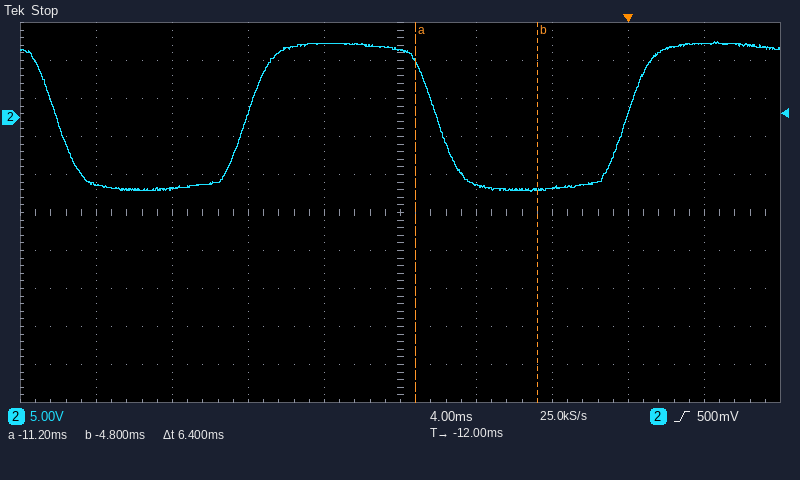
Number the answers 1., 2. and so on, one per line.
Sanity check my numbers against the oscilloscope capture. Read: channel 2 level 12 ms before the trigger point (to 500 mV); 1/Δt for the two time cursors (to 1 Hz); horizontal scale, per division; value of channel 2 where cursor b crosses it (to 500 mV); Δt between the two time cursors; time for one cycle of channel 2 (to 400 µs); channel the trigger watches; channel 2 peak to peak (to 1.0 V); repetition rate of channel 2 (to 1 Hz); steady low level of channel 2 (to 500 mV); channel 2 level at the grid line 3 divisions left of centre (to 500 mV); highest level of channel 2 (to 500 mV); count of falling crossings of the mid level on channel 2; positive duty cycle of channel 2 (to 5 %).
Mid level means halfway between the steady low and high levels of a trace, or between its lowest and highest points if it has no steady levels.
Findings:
1. 9.0 V
2. 156 Hz
3. 4 ms
4. -9.5 V
5. 6.4 ms
6. 20.0 ms
7. channel 2
8. 20.0 V
9. 50 Hz
10. -9.5 V
11. -9.5 V
12. 10.0 V
13. 2
14. 50 %
